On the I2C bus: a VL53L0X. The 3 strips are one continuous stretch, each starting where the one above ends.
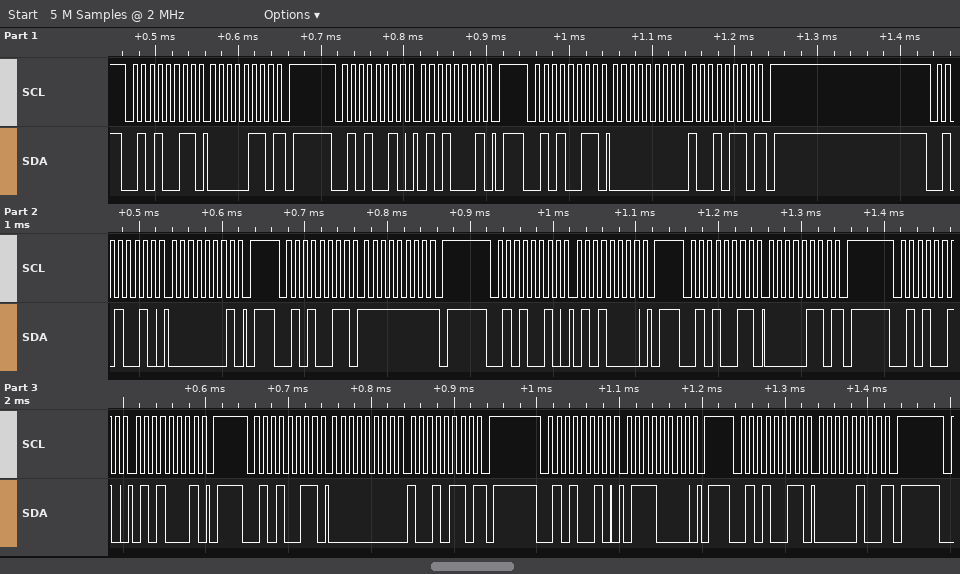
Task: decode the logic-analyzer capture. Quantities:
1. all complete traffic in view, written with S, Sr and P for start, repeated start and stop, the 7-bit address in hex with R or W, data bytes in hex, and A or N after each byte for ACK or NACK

S 29R A 06 N P S 29W A 51 A P S 29R A 00 A 96 N P S 29W A 01 A P S 29R A FF N P S 29W A 50 A P S 29R A 06 N P S 29W A 51 A P S 29R A 00 A 96 N P S 29W A 70 A P S 29R A 04 N P
